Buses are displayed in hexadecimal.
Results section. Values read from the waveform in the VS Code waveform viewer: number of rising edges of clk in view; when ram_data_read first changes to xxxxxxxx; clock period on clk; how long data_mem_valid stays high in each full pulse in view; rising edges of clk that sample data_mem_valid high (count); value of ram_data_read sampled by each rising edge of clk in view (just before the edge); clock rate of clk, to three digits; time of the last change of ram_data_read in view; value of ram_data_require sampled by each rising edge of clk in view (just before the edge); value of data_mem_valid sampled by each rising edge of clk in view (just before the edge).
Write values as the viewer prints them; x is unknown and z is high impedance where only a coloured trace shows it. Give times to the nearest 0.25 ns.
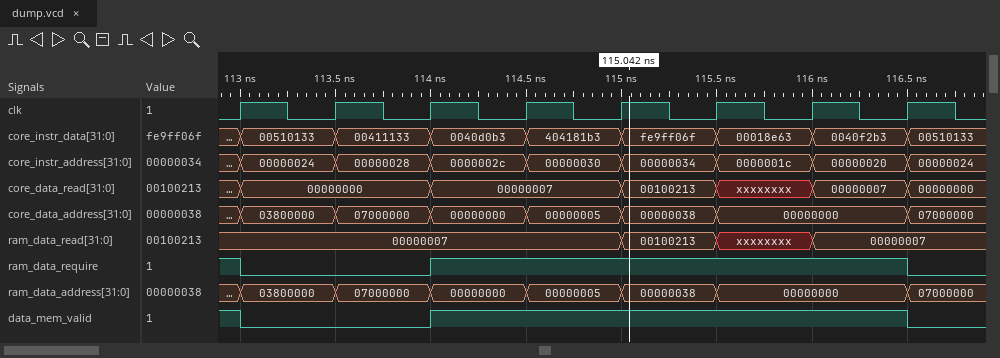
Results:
8
115.5 ns
0.5 ns
2.5 ns
6
00000007, 00000007, 00000007, 00000007, 00000007, 00100213, xxxxxxxx, 00000007
2.00 GHz
116 ns
1 0 0 1 1 1 1 1
1 0 0 1 1 1 1 1
